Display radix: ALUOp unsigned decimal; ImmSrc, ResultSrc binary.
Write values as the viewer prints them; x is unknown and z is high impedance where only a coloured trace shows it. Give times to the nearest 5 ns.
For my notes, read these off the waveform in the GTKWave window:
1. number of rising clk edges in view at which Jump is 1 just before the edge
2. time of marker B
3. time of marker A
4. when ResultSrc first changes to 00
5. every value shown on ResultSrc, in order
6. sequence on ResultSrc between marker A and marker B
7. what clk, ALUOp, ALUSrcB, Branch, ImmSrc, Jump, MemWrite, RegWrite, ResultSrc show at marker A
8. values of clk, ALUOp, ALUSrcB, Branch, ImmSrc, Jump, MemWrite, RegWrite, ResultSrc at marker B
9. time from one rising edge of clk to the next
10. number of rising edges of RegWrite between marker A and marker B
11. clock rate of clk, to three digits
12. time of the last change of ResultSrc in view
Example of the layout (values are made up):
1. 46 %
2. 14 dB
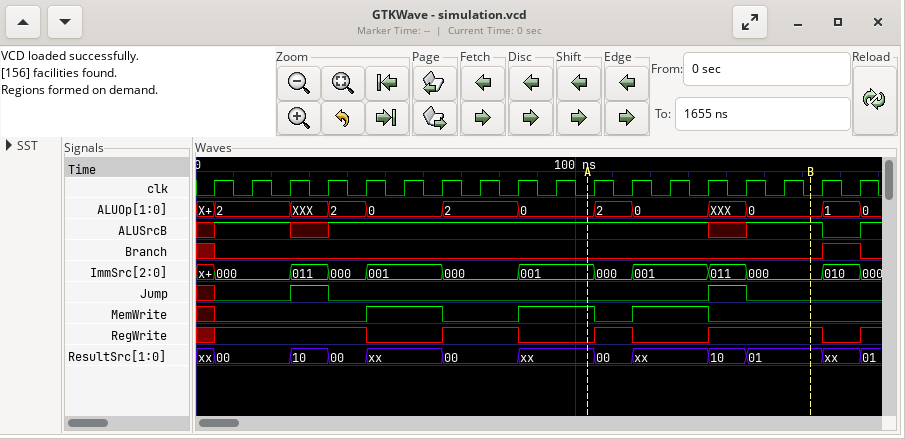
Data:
1. 2
2. 160 ns
3. 105 ns
4. 5 ns
5. xx, 00, 10, 00, xx, 00, xx, 00, xx, 10, 01, xx, 01
6. xx, 00, xx, 10, 01
7. clk=0, ALUOp=0, ALUSrcB=1, Branch=0, ImmSrc=001, Jump=0, MemWrite=1, RegWrite=0, ResultSrc=xx
8. clk=0, ALUOp=0, ALUSrcB=1, Branch=0, ImmSrc=000, Jump=0, MemWrite=0, RegWrite=1, ResultSrc=01
9. 10 ns
10. 2
11. 100 MHz
12. 175 ns
